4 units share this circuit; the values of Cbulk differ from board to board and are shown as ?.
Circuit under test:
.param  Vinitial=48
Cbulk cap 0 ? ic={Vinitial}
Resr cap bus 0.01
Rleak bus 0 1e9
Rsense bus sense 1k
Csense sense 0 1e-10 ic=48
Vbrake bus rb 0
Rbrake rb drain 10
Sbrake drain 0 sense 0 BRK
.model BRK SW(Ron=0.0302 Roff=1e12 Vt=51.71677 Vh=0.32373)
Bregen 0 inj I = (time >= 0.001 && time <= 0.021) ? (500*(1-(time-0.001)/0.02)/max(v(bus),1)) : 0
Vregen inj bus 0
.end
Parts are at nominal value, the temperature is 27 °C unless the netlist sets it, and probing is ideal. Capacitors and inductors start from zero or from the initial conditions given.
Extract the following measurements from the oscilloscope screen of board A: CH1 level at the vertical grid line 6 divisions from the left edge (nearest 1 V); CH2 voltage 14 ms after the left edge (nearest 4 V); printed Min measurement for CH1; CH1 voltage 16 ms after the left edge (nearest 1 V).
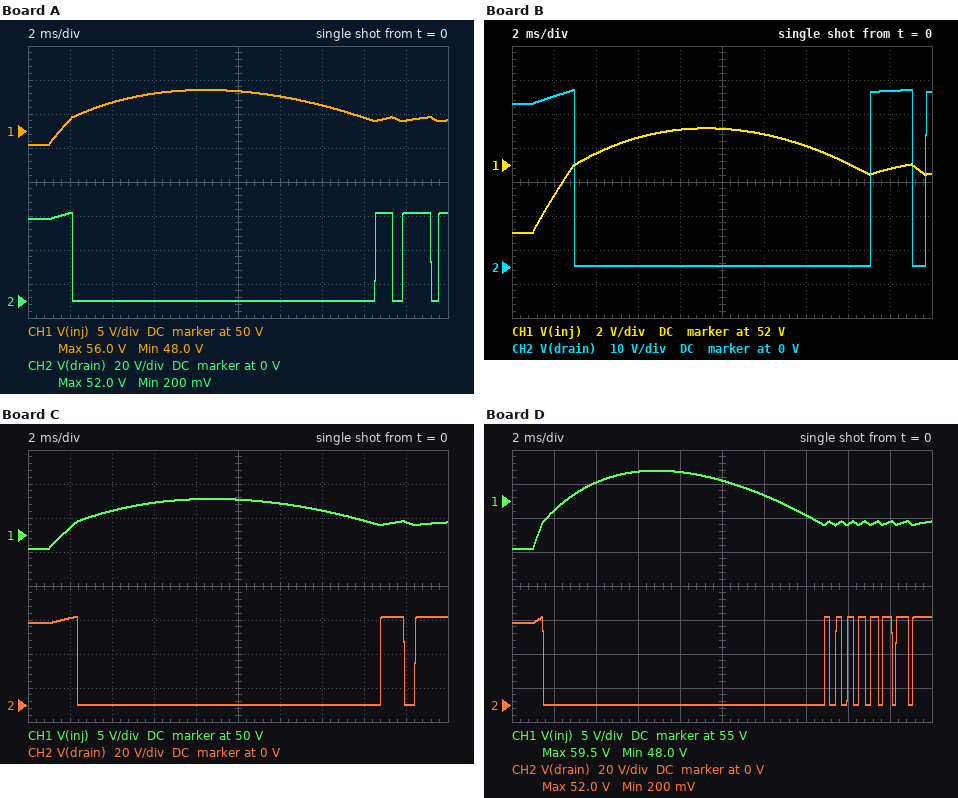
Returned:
55 V
0 V
48.0 V
52 V
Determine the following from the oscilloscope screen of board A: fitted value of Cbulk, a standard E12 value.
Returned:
2.7 mF
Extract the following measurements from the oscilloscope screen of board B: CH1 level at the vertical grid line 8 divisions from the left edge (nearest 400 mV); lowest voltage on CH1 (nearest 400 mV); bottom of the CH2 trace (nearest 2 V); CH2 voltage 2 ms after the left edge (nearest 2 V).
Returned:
52.0 V
48.0 V
0 V
50 V
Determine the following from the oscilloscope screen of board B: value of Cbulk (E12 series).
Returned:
4.7 mF
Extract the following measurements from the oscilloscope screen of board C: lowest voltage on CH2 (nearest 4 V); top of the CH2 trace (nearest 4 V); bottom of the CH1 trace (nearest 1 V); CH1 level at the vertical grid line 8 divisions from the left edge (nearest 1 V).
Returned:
0 V
52 V
48 V
52 V
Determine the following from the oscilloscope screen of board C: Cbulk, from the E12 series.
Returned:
3.3 mF
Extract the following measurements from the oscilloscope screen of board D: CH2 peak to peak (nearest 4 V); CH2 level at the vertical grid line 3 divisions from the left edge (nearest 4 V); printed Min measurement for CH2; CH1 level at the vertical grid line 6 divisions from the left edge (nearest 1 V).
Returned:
52 V
0 V
200 mV
56 V
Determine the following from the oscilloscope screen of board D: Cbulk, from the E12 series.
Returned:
1.2 mF
